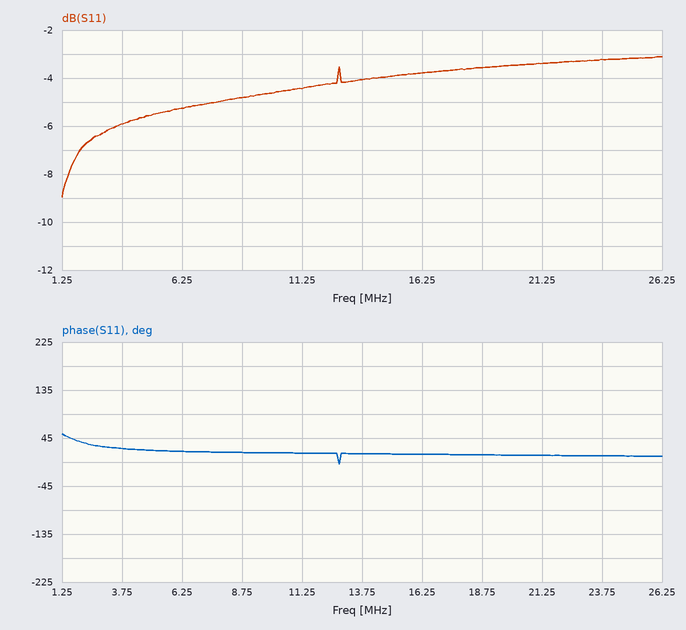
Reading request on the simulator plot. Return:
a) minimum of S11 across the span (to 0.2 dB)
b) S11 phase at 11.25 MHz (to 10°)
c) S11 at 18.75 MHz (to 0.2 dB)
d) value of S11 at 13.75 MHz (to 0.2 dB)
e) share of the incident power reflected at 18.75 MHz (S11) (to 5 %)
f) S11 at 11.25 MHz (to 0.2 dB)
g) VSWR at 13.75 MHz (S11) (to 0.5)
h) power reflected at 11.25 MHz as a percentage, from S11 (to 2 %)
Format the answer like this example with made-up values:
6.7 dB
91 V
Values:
-9.0 dB
20°
-3.6 dB
-4.0 dB
45 %
-4.4 dB
4.5
36 %
